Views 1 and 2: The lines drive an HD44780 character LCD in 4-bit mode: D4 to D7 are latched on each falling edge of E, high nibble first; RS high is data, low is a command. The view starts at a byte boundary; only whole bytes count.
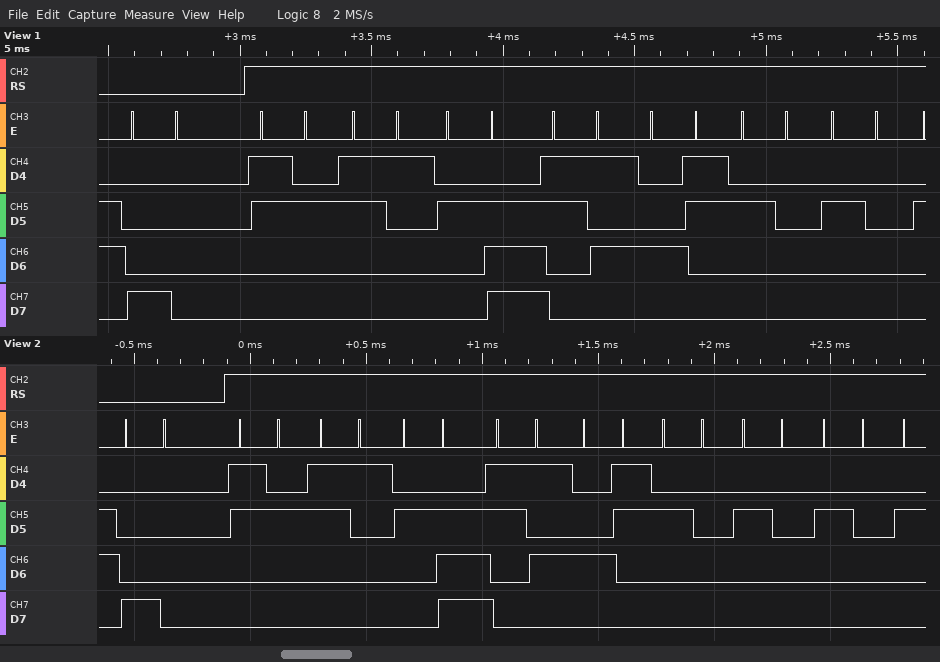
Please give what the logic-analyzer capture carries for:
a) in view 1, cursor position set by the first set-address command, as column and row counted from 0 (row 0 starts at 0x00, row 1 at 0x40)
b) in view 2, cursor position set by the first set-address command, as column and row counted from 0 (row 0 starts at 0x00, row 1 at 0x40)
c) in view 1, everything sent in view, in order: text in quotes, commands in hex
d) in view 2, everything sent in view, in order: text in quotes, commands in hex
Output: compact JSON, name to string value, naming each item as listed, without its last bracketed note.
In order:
{"in view 1, cursor position set by the first set-address command, as column and row counted from 0": "column 0, row 0", "in view 2, cursor position set by the first set-address command, as column and row counted from 0": "column 0, row 0", "in view 1, everything sent in view, in order: text in quotes, commands in hex": "0x80 \"21.5C  \"", "in view 2, everything sent in view, in order: text in quotes, commands in hex": "0x80 \"21.5C   \""}
